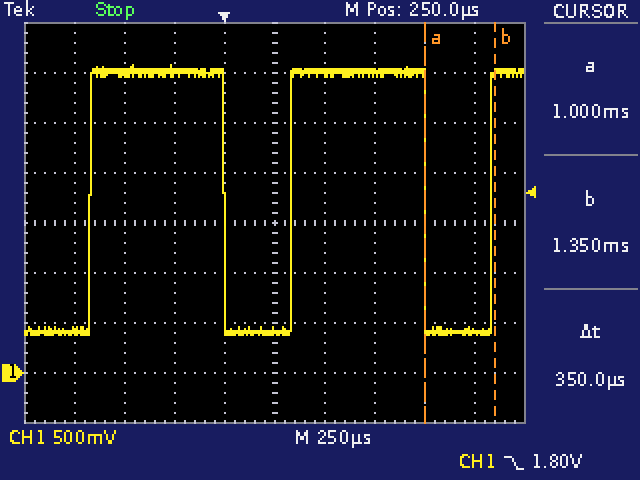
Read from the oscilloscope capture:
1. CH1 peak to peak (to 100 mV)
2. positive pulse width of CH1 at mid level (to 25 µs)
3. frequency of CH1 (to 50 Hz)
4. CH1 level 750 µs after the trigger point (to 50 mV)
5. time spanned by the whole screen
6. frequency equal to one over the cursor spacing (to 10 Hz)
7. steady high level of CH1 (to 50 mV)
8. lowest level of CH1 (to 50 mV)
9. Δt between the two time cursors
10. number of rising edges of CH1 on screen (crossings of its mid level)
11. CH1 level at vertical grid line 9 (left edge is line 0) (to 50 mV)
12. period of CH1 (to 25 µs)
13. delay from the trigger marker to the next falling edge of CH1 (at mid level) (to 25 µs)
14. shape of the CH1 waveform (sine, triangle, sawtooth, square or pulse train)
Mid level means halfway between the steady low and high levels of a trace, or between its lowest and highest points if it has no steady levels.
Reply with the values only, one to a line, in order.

2.70 V
675 µs
1.00 kHz
3.00 V
2.5 ms
2.86 kHz
3.00 V
400 mV
350 µs
3
400 mV
1.000 ms
1.000 ms
pulse train
